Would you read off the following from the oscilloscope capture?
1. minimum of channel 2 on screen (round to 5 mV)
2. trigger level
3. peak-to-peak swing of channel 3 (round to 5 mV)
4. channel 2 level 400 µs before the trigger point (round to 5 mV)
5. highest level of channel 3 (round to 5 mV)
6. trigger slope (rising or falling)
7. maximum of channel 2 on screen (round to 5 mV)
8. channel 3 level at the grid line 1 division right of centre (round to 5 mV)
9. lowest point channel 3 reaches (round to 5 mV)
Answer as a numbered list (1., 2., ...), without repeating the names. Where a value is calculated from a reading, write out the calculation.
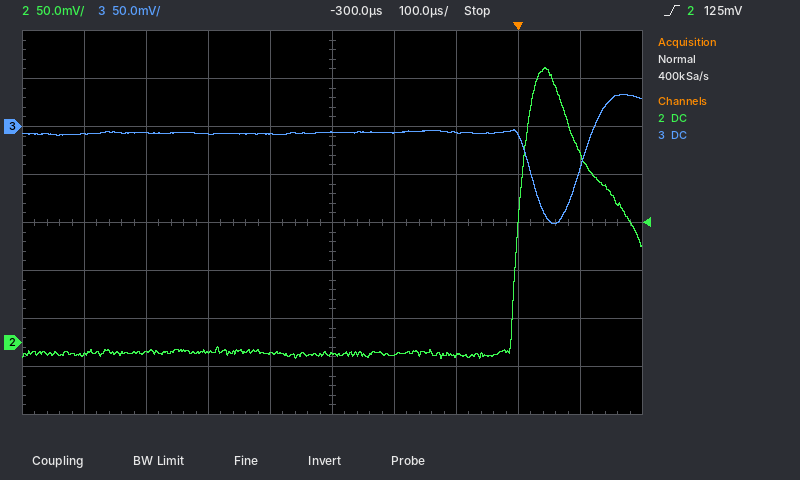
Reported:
1. -15 mV
2. 125 mV
3. 35 mV − (-100 mV) = 135 mV
4. -10 mV
5. 35 mV
6. rising
7. 285 mV
8. -5 mV
9. -100 mV
